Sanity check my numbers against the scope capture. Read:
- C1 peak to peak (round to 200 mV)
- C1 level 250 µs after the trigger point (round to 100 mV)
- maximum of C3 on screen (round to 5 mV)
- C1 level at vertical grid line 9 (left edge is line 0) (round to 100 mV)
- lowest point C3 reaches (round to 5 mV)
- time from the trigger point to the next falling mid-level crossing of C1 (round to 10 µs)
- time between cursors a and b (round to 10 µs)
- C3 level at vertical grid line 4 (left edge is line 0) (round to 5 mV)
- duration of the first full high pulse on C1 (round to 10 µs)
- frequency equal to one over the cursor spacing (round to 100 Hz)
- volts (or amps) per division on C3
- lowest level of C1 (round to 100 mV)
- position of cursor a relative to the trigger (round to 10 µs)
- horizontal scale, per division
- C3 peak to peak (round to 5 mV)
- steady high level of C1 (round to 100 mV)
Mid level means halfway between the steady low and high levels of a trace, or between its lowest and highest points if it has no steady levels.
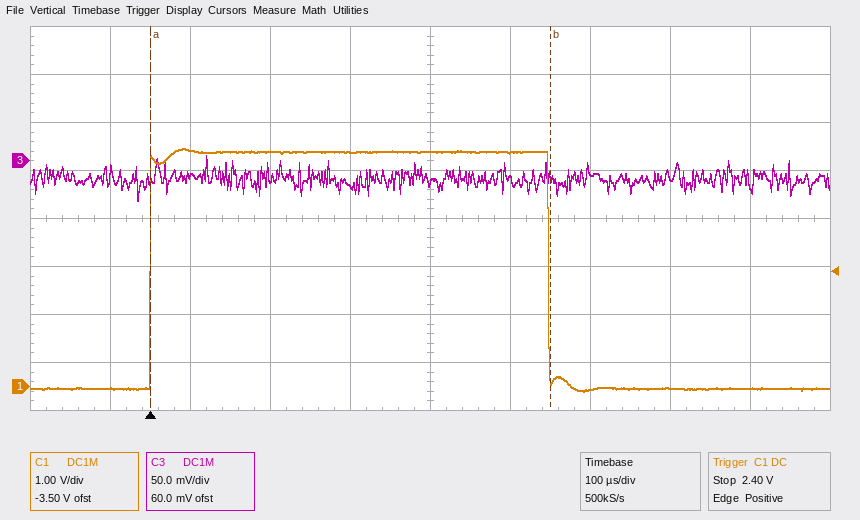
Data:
5.0 V
4.9 V
5 mV
0.0 V
-40 mV
500 µs
500 µs
-25 mV
500 µs
2.0 kHz
50 mV
-100 mV
0 µs
100 µs
45 mV
4.9 V
